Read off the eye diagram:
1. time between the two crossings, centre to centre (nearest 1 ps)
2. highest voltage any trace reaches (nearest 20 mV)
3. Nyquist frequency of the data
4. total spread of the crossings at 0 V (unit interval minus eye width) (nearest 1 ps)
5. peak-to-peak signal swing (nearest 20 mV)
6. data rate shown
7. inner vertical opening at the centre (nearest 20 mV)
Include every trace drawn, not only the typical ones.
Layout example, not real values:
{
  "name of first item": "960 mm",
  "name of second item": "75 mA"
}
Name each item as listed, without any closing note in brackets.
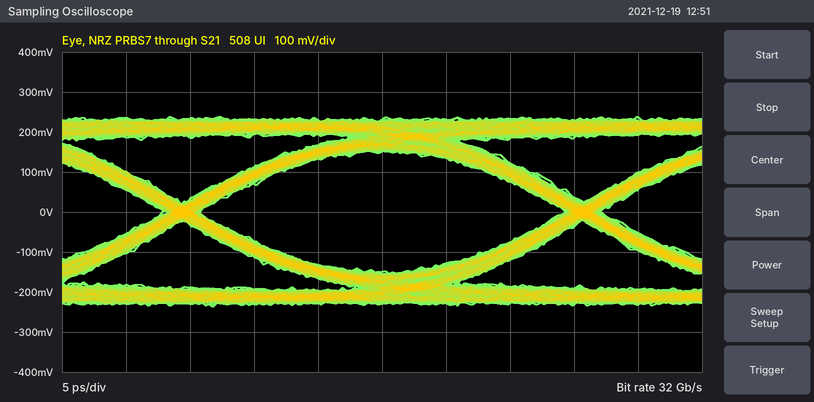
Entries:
{
  "time between the two crossings, centre to centre": "31 ps",
  "highest voltage any trace reaches": "240 mV",
  "Nyquist frequency of the data": "16 GHz",
  "total spread of the crossings at 0 V (unit interval minus eye width)": "3 ps",
  "peak-to-peak signal swing": "480 mV",
  "data rate shown": "32 Gb/s",
  "inner vertical opening at the centre": "300 mV"
}
